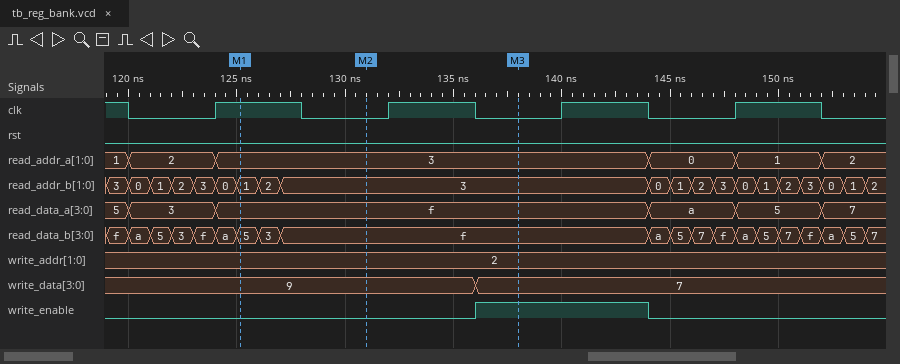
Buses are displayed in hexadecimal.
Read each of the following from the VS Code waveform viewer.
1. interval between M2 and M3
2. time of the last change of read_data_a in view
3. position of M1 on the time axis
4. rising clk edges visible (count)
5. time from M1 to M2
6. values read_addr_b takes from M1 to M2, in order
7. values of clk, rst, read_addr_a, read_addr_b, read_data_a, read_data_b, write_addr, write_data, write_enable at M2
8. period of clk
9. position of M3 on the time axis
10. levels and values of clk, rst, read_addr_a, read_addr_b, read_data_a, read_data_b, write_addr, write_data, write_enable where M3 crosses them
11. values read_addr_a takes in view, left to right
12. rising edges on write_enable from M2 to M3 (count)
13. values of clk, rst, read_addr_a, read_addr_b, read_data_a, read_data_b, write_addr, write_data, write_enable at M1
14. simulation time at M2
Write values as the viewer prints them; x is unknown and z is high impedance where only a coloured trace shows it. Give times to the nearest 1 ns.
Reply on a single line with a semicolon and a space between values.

7 ns; 152 ns; 125 ns; 4; 6 ns; 1, 2, 3; clk=0, rst=0, read_addr_a=3, read_addr_b=3, read_data_a=f, read_data_b=f, write_addr=2, write_data=9, write_enable=0; 8 ns; 138 ns; clk=0, rst=0, read_addr_a=3, read_addr_b=3, read_data_a=f, read_data_b=f, write_addr=2, write_data=7, write_enable=1; 1, 2, 3, 0, 1, 2; 1; clk=1, rst=0, read_addr_a=3, read_addr_b=1, read_data_a=f, read_data_b=5, write_addr=2, write_data=9, write_enable=0; 131 ns
